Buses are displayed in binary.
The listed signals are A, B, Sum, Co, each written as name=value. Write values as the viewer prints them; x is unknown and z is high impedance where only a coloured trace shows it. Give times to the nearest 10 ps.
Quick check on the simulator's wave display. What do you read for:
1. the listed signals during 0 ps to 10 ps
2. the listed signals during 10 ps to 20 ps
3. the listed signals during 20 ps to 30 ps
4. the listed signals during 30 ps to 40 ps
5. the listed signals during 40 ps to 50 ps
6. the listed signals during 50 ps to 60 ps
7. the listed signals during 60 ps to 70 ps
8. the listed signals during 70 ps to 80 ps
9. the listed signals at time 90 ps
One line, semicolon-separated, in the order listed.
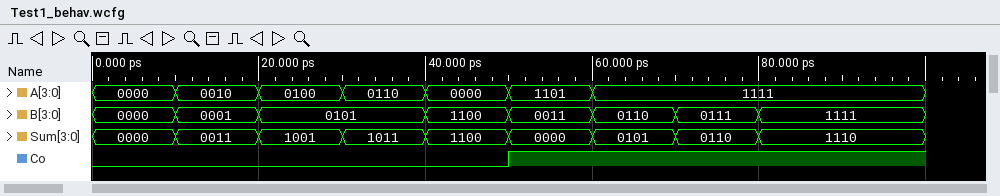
A=0000, B=0000, Sum=0000, Co=0; A=0010, B=0001, Sum=0011, Co=0; A=0100, B=0101, Sum=1001, Co=0; A=0110, B=0101, Sum=1011, Co=0; A=0000, B=1100, Sum=1100, Co=0; A=1101, B=0011, Sum=0000, Co=1; A=1111, B=0110, Sum=0101, Co=1; A=1111, B=0111, Sum=0110, Co=1; A=1111, B=1111, Sum=1110, Co=1
